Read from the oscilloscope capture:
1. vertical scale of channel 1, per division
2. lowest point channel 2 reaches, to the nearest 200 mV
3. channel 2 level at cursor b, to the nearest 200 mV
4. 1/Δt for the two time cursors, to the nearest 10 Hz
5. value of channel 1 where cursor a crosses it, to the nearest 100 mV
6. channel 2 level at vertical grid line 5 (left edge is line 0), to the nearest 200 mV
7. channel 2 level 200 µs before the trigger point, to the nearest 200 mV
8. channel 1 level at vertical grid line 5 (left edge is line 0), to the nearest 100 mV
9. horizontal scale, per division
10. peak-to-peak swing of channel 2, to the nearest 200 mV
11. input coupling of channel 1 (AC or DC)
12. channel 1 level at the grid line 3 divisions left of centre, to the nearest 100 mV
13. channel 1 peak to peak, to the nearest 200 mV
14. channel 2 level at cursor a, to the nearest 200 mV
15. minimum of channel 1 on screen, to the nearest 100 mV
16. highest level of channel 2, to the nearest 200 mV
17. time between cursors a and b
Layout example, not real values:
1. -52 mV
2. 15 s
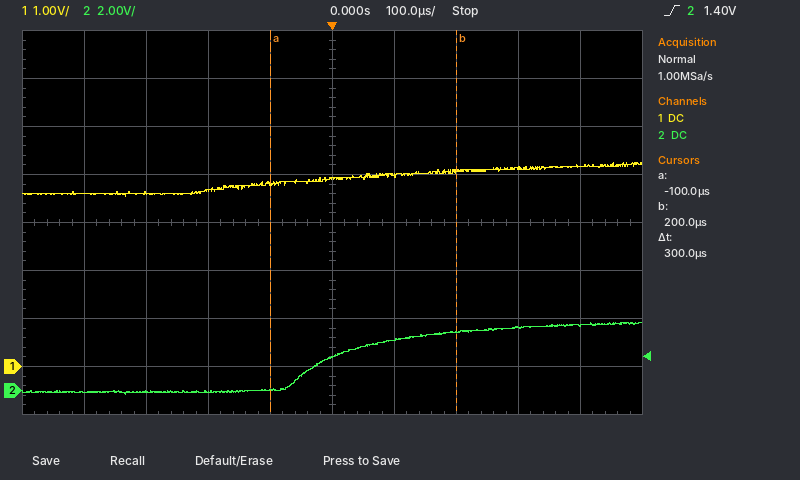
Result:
1. 1 V
2. -200 mV
3. 2.4 V
4. 3.33 kHz
5. 3.8 V
6. 1.4 V
7. 0.0 V
8. 3.9 V
9. 100 µs
10. 3.0 V
11. DC
12. 3.6 V
13. 800 mV
14. 0.0 V
15. 3.5 V
16. 2.8 V
17. 300 µs
